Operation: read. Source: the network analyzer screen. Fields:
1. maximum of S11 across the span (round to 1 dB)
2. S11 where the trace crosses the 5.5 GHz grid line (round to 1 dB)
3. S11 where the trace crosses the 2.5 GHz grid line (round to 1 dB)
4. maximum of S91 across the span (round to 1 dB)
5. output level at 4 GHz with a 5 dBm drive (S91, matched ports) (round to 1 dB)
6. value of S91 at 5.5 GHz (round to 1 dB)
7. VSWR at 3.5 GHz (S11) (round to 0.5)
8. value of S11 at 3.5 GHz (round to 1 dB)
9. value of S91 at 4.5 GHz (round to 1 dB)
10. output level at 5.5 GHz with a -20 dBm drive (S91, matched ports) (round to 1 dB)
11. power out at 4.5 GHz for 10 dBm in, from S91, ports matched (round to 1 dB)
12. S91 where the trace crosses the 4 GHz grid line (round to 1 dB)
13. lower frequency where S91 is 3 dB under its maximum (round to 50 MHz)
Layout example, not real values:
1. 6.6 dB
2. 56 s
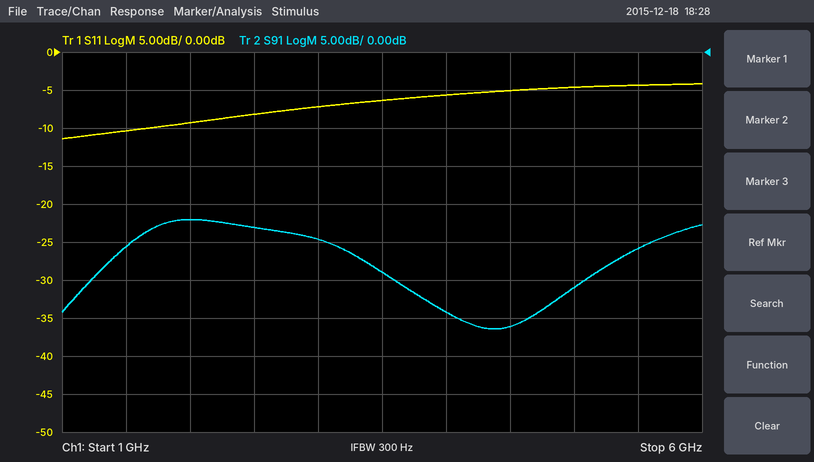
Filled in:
1. -4 dB
2. -4 dB
3. -8 dB
4. -22 dB
5. -29 dBm
6. -26 dB
7. 3.0
8. -6 dB
9. -36 dB
10. -46 dBm
11. -26 dBm
12. -34 dB
13. 1.55 GHz
